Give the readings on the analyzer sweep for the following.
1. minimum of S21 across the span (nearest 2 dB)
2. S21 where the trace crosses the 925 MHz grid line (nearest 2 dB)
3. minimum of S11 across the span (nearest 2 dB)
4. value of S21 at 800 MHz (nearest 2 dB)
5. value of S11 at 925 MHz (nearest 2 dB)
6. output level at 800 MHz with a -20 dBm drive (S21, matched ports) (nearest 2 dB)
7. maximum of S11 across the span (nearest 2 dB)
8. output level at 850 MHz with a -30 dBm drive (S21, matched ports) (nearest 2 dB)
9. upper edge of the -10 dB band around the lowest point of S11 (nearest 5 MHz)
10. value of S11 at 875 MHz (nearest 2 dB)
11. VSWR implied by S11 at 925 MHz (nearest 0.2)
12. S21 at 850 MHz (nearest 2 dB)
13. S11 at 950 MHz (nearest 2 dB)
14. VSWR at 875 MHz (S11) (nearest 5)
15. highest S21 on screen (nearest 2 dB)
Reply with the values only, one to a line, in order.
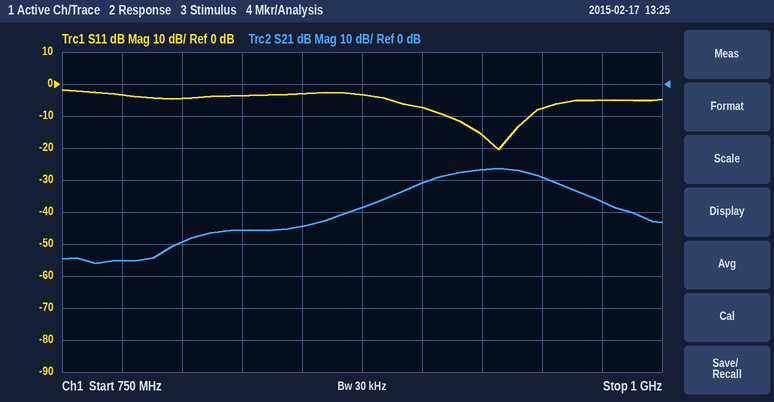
-56 dB
-26 dB
-20 dB
-50 dB
-16 dB
-70 dBm
-2 dB
-74 dBm
945 MHz
-4 dB
1.4
-44 dB
-8 dB
5
-26 dB
